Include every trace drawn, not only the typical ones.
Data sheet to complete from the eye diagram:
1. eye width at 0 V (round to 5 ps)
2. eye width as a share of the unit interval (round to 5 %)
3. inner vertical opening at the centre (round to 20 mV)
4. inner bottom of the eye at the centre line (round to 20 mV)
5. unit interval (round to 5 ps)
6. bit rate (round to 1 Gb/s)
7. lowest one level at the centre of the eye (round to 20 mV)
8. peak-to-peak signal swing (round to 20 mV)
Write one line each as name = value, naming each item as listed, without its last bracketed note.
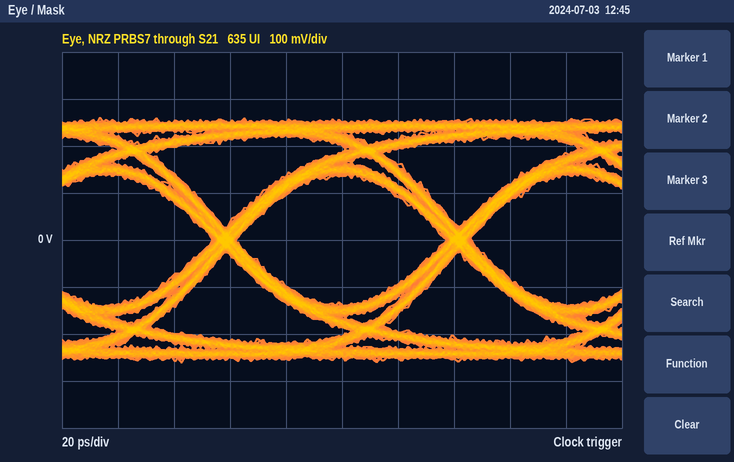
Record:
eye width at 0 V = 75 ps
eye width as a share of the unit interval = 90 %
inner vertical opening at the centre = 280 mV
inner bottom of the eye at the centre line = -140 mV
unit interval = 85 ps
bit rate = 12 Gb/s
lowest one level at the centre of the eye = 140 mV
peak-to-peak signal swing = 520 mV
